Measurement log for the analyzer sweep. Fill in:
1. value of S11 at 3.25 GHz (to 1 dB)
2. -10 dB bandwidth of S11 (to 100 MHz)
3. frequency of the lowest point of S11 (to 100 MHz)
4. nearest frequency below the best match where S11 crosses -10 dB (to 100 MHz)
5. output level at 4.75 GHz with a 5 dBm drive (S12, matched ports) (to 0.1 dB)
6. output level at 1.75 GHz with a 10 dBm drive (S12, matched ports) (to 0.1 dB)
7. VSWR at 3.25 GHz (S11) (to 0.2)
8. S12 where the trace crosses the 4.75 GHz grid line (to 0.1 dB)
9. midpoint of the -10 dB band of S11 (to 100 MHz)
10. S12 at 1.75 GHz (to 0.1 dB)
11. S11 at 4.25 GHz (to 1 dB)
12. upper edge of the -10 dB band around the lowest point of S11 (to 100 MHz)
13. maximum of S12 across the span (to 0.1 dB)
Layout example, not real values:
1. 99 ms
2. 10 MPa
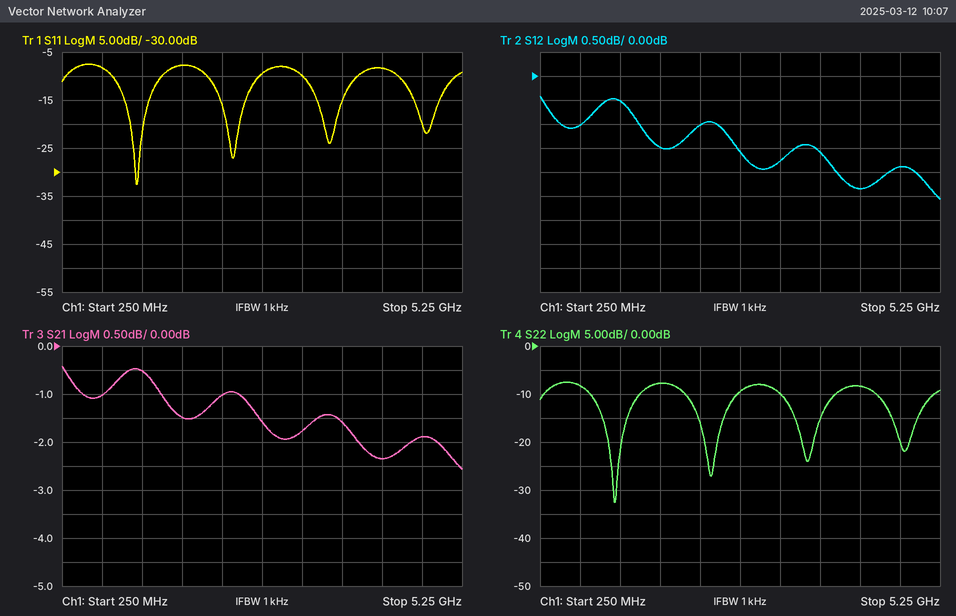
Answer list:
1. -10 dB
2. 600 MHz
3. 1.2 GHz
4. 900 MHz
5. 3.1 dBm
6. 8.5 dBm
7. 2.0
8. -1.9 dB
9. 1.2 GHz
10. -1.5 dB
11. -8 dB
12. 1.5 GHz
13. -0.4 dB
